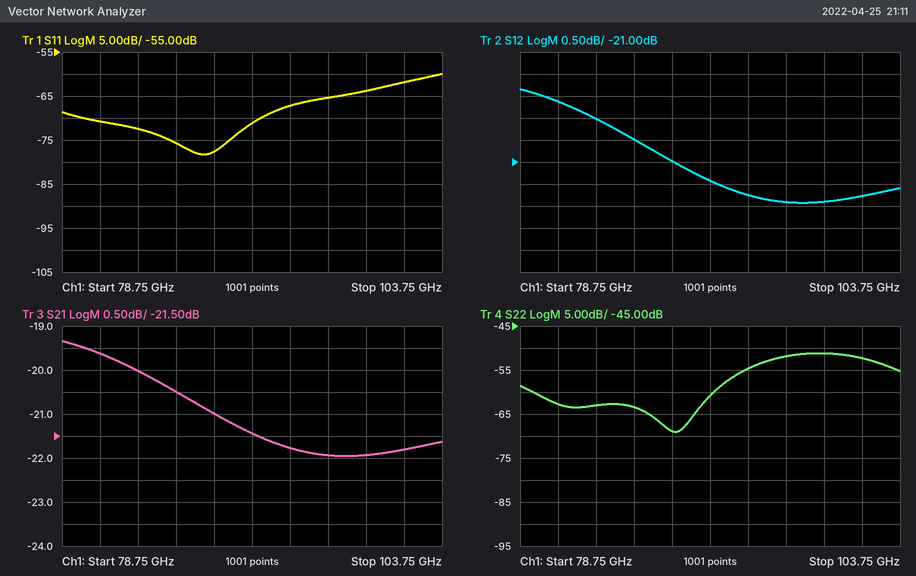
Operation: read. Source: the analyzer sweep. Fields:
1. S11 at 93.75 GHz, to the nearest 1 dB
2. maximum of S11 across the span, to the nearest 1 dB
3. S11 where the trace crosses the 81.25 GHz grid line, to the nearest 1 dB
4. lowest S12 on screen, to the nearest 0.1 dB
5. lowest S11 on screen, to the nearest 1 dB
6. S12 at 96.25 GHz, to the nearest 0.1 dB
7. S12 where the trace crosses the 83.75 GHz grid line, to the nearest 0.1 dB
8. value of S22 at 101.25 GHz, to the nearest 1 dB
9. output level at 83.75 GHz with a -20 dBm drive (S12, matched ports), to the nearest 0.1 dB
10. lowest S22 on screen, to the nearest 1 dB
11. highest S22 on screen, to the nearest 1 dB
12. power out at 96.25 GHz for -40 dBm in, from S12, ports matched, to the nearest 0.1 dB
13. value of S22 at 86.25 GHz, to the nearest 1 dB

-67 dB
-60 dB
-71 dB
-21.9 dB
-78 dB
-21.9 dB
-20.0 dB
-52 dB
-40.0 dBm
-69 dB
-51 dB
-61.9 dBm
-63 dB
